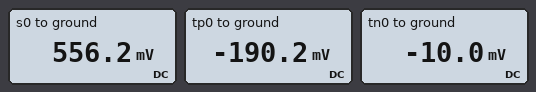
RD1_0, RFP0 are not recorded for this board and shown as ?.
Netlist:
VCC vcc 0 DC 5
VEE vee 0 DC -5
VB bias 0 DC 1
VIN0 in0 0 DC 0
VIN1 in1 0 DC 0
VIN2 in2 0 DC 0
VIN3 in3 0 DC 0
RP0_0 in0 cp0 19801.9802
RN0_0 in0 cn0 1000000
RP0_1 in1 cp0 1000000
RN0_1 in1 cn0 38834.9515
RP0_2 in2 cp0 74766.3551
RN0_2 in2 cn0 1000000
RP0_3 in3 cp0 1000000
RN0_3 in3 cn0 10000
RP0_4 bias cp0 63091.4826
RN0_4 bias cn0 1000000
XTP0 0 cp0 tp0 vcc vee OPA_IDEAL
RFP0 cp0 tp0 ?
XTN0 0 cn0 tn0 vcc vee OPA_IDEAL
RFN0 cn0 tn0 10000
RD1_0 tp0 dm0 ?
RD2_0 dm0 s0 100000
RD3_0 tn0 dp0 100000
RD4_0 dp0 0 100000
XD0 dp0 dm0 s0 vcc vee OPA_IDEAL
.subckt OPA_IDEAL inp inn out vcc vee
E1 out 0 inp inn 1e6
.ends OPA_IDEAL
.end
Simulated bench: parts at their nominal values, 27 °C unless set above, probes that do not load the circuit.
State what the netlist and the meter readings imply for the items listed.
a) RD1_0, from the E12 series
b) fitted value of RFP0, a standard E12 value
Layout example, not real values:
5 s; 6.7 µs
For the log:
33 kΩ; 12 kΩ
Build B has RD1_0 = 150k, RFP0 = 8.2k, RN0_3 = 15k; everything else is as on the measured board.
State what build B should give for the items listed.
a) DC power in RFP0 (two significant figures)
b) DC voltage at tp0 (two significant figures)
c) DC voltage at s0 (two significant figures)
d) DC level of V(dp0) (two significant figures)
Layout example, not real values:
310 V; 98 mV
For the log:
2.1 µW; -130 mV; 78 mV; -5.0 mV
